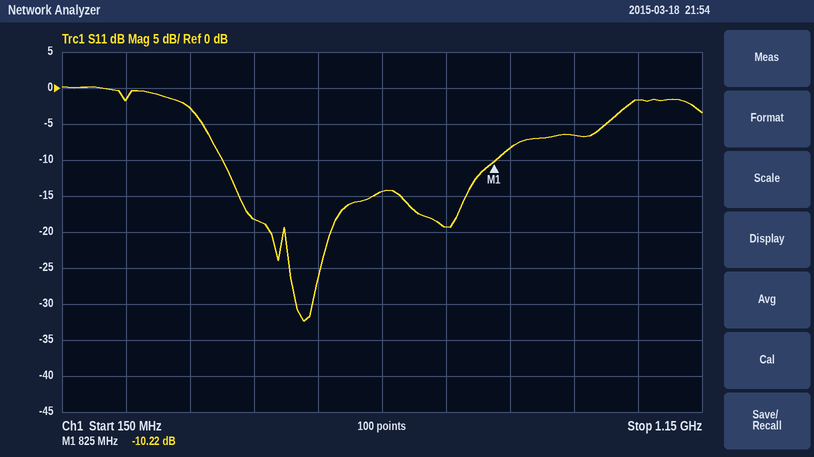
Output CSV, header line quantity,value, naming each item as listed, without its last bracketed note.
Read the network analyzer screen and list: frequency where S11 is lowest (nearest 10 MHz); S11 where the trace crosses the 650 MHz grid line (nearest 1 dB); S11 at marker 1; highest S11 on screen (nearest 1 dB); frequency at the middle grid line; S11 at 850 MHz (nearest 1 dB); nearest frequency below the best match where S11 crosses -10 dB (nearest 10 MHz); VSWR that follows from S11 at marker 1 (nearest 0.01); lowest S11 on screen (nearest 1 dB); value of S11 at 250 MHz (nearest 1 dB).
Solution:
quantity,value
frequency where S11 is lowest,530 MHz
S11 where the trace crosses the 650 MHz grid line,-14 dB
S11 at marker 1,-10.22 dB
highest S11 on screen,0 dB
frequency at the middle grid line,650 MHz
S11 at 850 MHz,-8 dB
nearest frequency below the best match where S11 crosses -10 dB,400 MHz
VSWR that follows from S11 at marker 1,1.89
lowest S11 on screen,-32 dB
value of S11 at 250 MHz,-2 dB
